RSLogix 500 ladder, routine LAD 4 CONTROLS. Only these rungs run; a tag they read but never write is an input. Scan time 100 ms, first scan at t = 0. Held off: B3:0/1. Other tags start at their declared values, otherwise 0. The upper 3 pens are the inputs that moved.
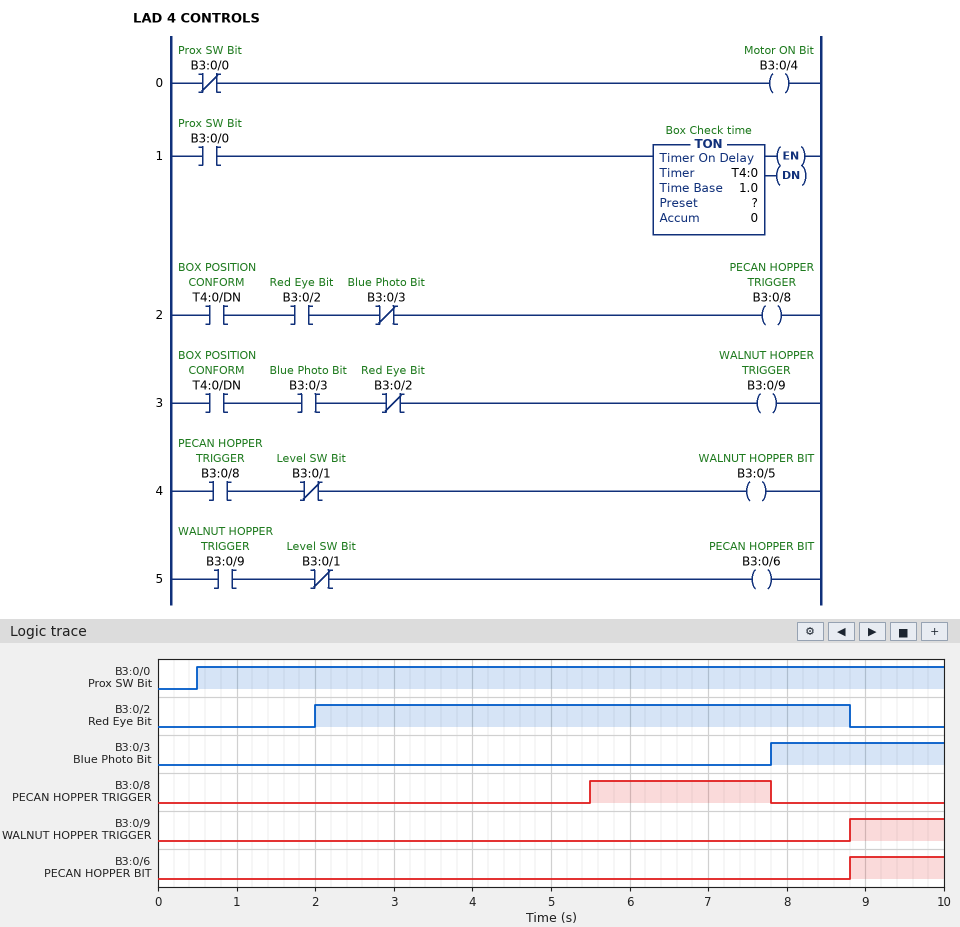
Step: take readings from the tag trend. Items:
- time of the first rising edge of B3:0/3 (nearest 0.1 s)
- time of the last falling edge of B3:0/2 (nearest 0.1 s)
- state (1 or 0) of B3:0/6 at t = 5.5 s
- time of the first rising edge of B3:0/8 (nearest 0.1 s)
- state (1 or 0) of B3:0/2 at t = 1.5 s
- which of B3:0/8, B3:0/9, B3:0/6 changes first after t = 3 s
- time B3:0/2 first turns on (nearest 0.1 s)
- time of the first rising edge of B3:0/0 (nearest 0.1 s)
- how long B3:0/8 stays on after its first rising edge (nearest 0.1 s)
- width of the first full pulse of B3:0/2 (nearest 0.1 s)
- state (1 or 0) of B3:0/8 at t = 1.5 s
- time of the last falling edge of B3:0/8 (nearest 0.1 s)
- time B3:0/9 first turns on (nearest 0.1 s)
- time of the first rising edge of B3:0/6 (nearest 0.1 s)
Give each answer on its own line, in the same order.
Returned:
7.8 s
8.8 s
0
5.5 s
0
B3:0/8
2.0 s
0.5 s
2.3 s
6.8 s
0
7.8 s
8.8 s
8.8 s
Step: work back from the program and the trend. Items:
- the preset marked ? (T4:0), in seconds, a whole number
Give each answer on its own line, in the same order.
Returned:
5 s
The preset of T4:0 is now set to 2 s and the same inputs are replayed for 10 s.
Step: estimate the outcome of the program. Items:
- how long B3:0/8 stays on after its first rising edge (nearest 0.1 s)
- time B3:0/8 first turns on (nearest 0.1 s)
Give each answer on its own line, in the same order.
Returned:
5.3 s
2.5 s
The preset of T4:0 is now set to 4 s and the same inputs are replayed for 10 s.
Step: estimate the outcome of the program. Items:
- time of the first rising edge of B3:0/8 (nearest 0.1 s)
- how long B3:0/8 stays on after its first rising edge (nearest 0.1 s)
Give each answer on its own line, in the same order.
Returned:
4.5 s
3.3 s
